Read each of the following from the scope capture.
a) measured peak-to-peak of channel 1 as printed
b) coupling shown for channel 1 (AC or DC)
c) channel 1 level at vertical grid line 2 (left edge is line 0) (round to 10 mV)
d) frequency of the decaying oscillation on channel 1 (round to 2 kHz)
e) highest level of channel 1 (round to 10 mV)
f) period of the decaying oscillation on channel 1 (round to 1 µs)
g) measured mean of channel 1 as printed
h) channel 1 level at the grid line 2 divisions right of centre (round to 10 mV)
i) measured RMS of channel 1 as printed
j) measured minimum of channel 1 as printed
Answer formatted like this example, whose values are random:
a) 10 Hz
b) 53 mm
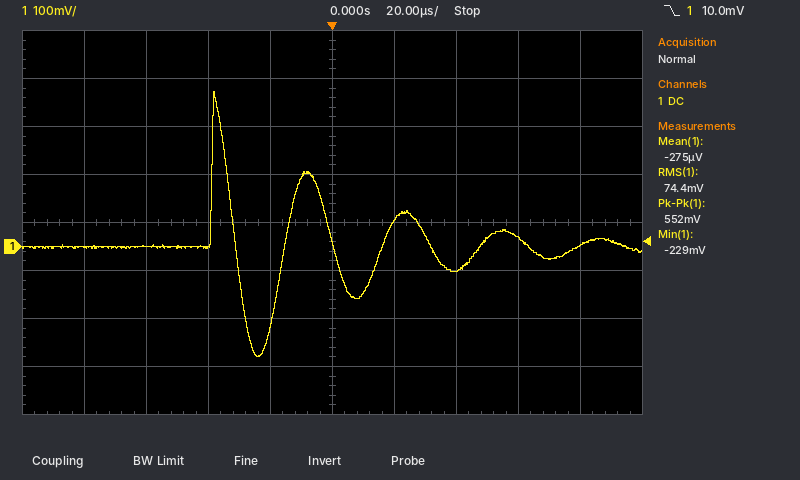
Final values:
a) 552 mV
b) DC
c) 0 mV
d) 32 kHz
e) 320 mV
f) 31 µs
g) -275 µV
h) -50 mV
i) 74.4 mV
j) -229 mV
